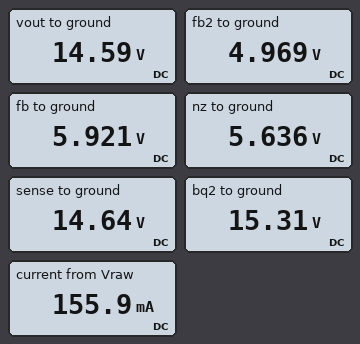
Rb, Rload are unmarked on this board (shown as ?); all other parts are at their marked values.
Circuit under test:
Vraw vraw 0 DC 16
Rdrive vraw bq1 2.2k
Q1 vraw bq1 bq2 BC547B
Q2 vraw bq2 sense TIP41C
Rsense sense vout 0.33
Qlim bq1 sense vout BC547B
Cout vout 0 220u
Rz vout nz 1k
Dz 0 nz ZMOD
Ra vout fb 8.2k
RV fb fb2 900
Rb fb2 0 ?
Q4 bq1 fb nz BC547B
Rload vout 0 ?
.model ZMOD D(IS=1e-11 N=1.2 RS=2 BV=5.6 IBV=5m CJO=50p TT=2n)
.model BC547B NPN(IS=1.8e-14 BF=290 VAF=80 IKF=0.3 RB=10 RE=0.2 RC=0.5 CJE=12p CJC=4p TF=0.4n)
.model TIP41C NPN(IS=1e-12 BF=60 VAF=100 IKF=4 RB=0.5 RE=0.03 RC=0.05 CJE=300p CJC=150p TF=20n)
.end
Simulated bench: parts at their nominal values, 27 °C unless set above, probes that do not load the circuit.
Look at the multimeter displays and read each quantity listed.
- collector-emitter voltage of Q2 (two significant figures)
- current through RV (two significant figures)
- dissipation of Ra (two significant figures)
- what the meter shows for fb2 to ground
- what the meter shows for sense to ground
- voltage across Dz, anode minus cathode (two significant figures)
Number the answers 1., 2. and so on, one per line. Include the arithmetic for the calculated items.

1. 16 V - 14.64 V = 1.4 V
2. (5.921 V - 4.969 V) / 900 Ω = 1.1 mA
3. (14.59 V - 5.921 V)^2 / 8.2 kΩ = 9.2 mW
4. 4.969 V
5. 14.64 V
6. 0 V - 5.636 V = -5.6 V
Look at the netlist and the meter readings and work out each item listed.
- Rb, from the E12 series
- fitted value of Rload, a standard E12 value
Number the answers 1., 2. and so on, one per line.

1. 4.7 kΩ
2. 100 Ω
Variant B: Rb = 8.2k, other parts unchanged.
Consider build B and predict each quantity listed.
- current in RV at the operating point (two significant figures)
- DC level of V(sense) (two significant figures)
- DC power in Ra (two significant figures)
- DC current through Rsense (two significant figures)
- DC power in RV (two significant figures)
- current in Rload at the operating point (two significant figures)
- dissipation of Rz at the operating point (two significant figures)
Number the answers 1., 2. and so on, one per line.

1. 690 µA
2. 12 V
3. 3.9 mW
4. 130 mA
5. 430 µW
6. 120 mA
7. 40 mW
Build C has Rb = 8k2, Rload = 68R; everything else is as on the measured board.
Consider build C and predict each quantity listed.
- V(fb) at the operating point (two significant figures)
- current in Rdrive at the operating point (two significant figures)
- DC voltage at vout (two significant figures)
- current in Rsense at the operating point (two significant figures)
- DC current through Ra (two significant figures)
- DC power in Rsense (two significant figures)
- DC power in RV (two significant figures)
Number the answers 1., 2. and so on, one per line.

1. 6.3 V
2. 1.2 mA
3. 12 V
4. 180 mA
5. 690 µA
6. 11 mW
7. 430 µW
